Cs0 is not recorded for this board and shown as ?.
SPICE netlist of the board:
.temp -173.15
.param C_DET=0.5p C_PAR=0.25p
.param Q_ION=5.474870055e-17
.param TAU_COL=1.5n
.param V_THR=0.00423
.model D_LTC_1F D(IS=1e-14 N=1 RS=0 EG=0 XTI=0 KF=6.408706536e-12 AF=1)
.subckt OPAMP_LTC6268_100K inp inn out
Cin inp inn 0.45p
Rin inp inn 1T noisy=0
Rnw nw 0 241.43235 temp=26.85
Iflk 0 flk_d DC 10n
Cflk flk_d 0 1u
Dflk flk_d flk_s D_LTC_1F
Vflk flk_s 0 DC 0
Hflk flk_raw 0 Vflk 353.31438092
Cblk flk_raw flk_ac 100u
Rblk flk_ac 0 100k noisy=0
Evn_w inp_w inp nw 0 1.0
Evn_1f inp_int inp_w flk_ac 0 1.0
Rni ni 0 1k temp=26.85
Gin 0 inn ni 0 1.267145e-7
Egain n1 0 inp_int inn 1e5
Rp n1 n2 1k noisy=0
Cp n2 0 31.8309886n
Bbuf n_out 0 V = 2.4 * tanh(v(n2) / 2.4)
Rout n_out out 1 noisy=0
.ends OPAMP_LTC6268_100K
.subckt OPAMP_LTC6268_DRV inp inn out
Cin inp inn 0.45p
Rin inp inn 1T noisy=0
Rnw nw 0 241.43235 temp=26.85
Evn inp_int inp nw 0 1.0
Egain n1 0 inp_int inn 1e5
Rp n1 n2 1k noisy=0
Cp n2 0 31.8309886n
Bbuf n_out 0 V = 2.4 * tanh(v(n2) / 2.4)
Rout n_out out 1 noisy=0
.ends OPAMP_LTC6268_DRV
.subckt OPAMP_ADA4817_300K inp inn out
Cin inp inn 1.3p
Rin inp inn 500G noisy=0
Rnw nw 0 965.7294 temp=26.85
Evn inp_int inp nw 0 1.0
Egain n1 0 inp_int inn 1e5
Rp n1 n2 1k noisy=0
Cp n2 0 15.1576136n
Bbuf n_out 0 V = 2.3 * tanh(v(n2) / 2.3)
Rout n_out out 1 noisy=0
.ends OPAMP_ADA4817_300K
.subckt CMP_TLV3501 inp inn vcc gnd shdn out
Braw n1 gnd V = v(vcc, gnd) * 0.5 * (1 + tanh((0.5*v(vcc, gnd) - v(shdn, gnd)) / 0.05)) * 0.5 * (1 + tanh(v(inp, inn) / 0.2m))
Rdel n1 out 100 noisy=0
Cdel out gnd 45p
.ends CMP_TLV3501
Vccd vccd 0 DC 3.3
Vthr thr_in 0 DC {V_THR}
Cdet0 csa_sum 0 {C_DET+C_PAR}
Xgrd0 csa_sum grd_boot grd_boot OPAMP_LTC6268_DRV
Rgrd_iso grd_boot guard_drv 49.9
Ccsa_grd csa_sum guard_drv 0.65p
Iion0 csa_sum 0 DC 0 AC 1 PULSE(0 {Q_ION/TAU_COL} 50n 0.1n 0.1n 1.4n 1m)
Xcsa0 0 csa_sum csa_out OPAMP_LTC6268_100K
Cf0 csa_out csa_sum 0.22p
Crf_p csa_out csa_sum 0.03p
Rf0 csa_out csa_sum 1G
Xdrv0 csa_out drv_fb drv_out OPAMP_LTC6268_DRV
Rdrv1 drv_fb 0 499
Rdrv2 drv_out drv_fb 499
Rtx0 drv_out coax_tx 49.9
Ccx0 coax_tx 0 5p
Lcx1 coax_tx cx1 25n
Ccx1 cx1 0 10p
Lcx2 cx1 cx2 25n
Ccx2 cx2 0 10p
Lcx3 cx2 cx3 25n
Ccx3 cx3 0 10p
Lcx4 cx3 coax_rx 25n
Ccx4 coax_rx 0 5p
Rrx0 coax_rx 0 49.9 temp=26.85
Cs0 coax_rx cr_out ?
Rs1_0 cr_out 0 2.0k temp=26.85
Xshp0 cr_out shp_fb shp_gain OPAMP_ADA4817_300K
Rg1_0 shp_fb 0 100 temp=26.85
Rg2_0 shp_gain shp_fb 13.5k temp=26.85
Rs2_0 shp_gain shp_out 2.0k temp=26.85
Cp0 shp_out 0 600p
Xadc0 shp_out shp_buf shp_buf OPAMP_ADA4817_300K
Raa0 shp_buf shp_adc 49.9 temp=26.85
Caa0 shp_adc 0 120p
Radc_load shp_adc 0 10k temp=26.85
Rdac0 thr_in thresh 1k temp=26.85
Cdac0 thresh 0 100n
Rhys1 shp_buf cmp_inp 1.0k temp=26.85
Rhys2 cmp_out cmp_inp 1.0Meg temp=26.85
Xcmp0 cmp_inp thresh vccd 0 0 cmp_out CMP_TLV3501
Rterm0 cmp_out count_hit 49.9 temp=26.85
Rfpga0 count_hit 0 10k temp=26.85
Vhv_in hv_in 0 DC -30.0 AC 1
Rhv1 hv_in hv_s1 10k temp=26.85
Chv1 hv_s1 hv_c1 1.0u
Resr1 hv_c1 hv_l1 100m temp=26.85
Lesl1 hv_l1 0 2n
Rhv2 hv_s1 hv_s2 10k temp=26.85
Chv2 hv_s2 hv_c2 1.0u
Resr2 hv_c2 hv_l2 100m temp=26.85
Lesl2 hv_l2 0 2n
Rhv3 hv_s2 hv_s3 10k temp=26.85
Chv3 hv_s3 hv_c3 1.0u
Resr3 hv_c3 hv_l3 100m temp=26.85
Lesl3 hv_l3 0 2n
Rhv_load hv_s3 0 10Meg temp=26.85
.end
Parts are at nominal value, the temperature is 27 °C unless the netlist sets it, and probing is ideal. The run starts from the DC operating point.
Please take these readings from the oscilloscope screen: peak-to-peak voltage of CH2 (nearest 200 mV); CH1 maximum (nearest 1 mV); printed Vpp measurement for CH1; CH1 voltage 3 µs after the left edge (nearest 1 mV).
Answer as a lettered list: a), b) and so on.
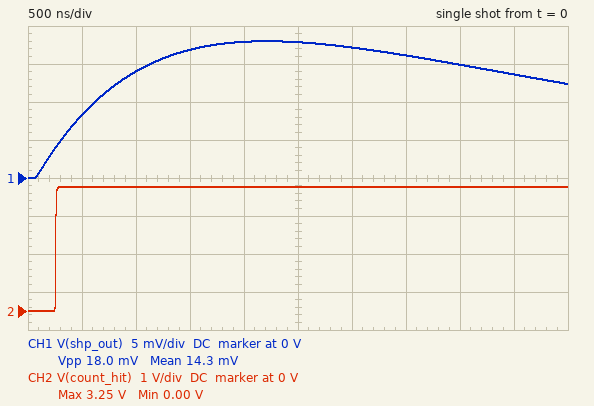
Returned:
a) 3.2 V
b) 18 mV
c) 18.0 mV
d) 17 mV
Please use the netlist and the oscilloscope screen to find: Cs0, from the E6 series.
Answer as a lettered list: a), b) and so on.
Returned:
a) 2.2 nF
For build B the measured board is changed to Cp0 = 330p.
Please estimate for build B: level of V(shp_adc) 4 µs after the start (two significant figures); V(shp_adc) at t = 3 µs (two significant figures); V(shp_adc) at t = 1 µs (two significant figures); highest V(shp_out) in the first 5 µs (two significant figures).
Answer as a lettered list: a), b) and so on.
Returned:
a) 14 mV
b) 17 mV
c) 19 mV
d) 21 mV
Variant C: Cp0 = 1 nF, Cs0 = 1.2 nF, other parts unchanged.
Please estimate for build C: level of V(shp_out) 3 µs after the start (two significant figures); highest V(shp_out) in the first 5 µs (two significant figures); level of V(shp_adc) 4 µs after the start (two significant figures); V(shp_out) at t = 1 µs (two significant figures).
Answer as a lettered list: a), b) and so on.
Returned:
a) 11 mV
b) 12 mV
c) 9.5 mV
d) 8.9 mV
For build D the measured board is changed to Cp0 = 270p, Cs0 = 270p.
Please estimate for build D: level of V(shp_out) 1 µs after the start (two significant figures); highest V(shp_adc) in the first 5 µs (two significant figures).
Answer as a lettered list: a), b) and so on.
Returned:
a) 9.1 mV
b) 11 mV
